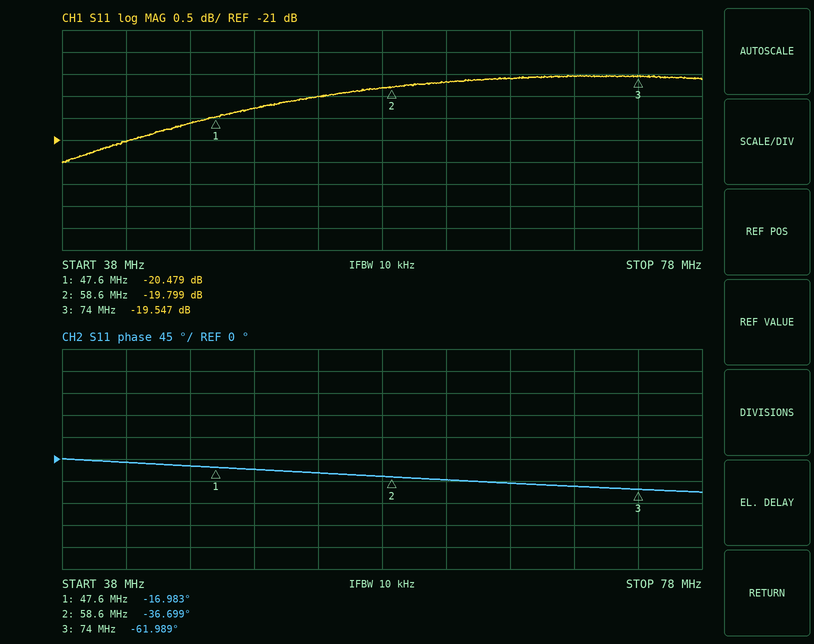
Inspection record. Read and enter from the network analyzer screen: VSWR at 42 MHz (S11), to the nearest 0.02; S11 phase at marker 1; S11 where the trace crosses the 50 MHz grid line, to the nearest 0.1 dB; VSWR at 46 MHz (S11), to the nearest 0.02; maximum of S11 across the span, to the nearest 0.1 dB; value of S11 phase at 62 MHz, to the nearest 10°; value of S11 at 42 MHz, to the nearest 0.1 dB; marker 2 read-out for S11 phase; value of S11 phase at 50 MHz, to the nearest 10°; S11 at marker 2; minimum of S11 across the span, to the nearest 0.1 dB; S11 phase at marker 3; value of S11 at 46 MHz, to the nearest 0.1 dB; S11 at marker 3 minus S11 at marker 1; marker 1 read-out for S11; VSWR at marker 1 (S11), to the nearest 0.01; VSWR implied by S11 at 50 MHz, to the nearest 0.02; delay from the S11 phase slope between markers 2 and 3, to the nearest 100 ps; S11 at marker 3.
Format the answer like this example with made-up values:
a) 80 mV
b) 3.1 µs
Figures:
a) 1.20
b) -16.983°
c) -20.3 dB
d) 1.20
e) -19.5 dB
f) -40°
g) -21.0 dB
h) -36.699°
i) -20°
j) -19.799 dB
k) -21.5 dB
l) -61.989°
m) -20.6 dB
n) 0.932 dB
o) -20.479 dB
p) 1.21
q) 1.22
r) 4.6 ns
s) -19.547 dB
